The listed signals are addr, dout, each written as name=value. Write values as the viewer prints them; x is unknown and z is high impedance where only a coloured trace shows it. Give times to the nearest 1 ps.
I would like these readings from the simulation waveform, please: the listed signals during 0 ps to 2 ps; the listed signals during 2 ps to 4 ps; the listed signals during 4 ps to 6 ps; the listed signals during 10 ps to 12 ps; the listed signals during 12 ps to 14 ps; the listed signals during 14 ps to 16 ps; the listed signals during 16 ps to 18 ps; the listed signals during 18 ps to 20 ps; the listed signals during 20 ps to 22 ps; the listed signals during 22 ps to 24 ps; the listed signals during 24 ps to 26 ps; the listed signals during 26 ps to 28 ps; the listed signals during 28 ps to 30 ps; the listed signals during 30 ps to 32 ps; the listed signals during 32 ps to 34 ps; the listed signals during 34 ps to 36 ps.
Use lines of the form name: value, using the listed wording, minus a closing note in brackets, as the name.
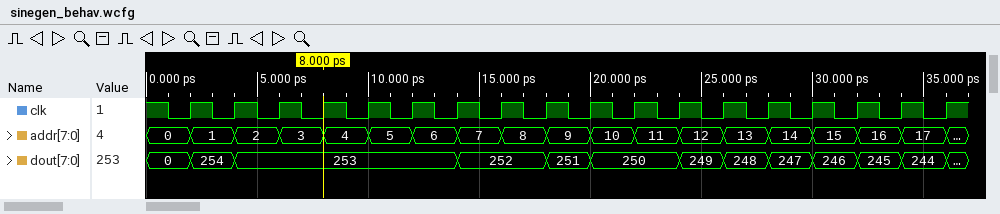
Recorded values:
the listed signals during 0 ps to 2 ps: addr=0, dout=0
the listed signals during 2 ps to 4 ps: addr=1, dout=254
the listed signals during 4 ps to 6 ps: addr=2, dout=253
the listed signals during 10 ps to 12 ps: addr=5, dout=253
the listed signals during 12 ps to 14 ps: addr=6, dout=253
the listed signals during 14 ps to 16 ps: addr=7, dout=252
the listed signals during 16 ps to 18 ps: addr=8, dout=252
the listed signals during 18 ps to 20 ps: addr=9, dout=251
the listed signals during 20 ps to 22 ps: addr=10, dout=250
the listed signals during 22 ps to 24 ps: addr=11, dout=250
the listed signals during 24 ps to 26 ps: addr=12, dout=249
the listed signals during 26 ps to 28 ps: addr=13, dout=248
the listed signals during 28 ps to 30 ps: addr=14, dout=247
the listed signals during 30 ps to 32 ps: addr=15, dout=246
the listed signals during 32 ps to 34 ps: addr=16, dout=245
the listed signals during 34 ps to 36 ps: addr=17, dout=244
